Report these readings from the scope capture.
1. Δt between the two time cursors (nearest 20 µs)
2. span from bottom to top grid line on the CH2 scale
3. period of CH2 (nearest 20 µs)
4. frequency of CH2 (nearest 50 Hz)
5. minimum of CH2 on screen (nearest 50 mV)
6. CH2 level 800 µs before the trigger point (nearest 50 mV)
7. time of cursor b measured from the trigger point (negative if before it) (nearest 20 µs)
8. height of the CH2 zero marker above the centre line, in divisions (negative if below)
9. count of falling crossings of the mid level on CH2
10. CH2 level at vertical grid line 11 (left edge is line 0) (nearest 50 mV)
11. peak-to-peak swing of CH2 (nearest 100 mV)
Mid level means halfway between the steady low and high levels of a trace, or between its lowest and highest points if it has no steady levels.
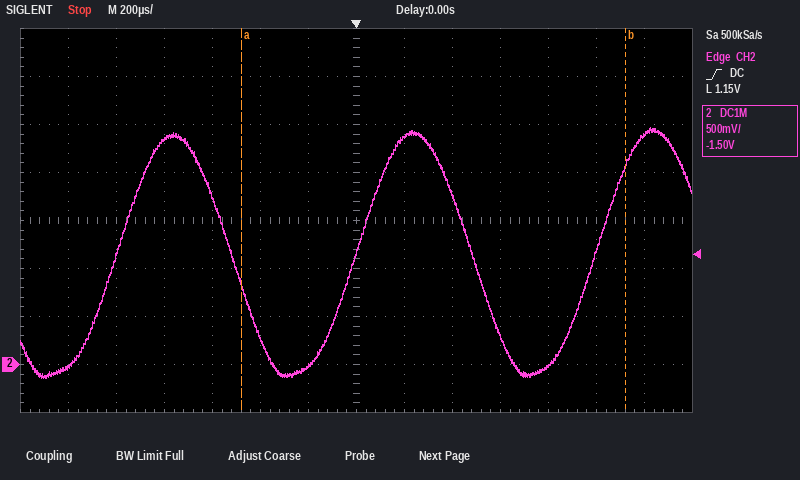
1.60 ms
4 V
1.00 ms
1.00 kHz
-150 mV
2.35 V
+1.12 ms
-3.0 div
2
0 mV
2.60 V
